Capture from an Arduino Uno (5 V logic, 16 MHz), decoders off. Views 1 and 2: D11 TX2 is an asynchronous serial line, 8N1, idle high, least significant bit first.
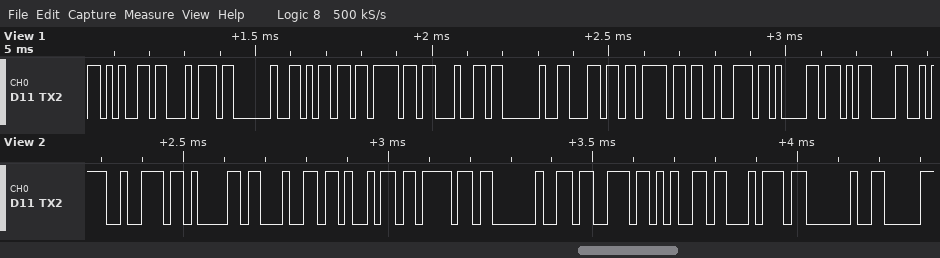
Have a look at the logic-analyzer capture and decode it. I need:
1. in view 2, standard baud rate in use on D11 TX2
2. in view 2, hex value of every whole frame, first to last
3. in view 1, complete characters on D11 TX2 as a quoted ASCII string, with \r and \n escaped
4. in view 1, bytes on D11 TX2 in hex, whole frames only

57600 baud
72 61 64 69 6F 20 73 65 74 20
"et mod lora\r"
0x65 0x74 0x20 0x6D 0x6F 0x64 0x20 0x6C 0x6F 0x72 0x61 0x0D
